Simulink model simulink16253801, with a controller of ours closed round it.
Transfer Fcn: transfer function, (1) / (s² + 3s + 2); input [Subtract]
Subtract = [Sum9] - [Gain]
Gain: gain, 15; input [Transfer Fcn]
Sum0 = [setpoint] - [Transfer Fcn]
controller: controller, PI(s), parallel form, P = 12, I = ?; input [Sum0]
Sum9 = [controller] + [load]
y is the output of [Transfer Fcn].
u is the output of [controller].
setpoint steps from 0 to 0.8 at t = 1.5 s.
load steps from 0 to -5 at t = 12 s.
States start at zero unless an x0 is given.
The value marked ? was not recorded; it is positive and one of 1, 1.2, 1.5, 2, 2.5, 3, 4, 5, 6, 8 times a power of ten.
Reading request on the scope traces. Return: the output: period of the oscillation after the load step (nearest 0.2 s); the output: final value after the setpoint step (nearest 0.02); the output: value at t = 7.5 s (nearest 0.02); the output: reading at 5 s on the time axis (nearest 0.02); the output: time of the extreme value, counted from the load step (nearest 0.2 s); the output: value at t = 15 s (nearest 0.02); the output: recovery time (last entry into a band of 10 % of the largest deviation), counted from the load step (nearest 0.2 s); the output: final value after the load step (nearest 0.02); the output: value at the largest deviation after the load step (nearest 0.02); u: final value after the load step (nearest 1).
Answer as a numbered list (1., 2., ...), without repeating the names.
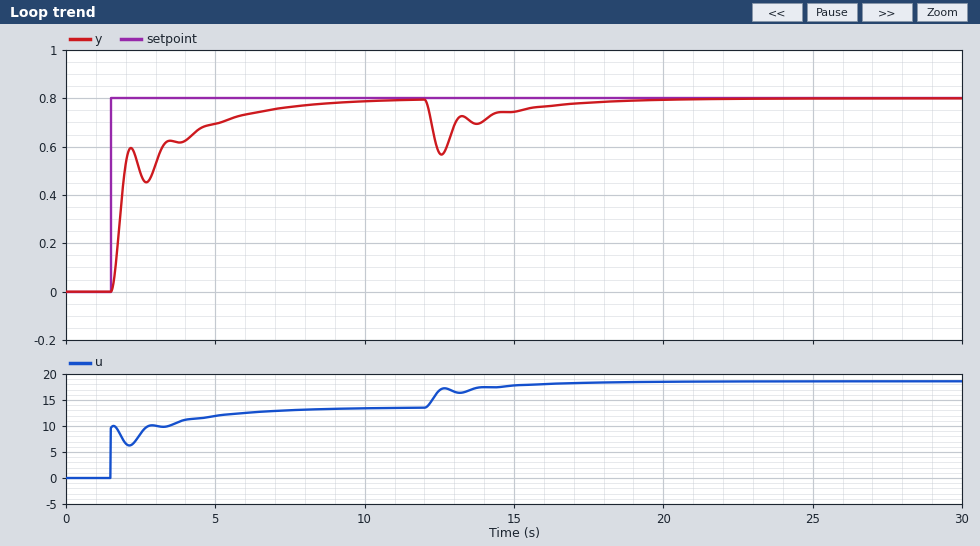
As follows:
1. 1.2 s
2. 0.80
3. 0.76
4. 0.70
5. 0.6 s
6. 0.74
7. 5.0 s
8. 0.80
9. 0.56
10. 19
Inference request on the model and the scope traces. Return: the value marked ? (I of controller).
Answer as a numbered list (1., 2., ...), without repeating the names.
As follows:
1. 12
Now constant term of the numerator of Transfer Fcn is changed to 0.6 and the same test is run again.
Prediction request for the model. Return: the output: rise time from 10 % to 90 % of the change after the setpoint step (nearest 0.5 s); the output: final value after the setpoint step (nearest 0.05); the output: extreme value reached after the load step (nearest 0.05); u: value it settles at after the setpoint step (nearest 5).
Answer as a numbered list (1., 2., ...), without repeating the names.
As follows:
1. 4.0 s
2. 0.80
3. 0.60
4. 15
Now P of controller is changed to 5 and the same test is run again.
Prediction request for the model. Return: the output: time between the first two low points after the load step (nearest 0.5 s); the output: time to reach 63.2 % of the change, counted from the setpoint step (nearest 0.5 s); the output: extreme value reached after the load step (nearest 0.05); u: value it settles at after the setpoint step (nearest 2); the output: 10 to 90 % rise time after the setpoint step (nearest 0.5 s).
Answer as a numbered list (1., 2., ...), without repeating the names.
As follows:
1. 1.5 s
2. 1.5 s
3. 0.50
4. 14
5. 3.5 s
